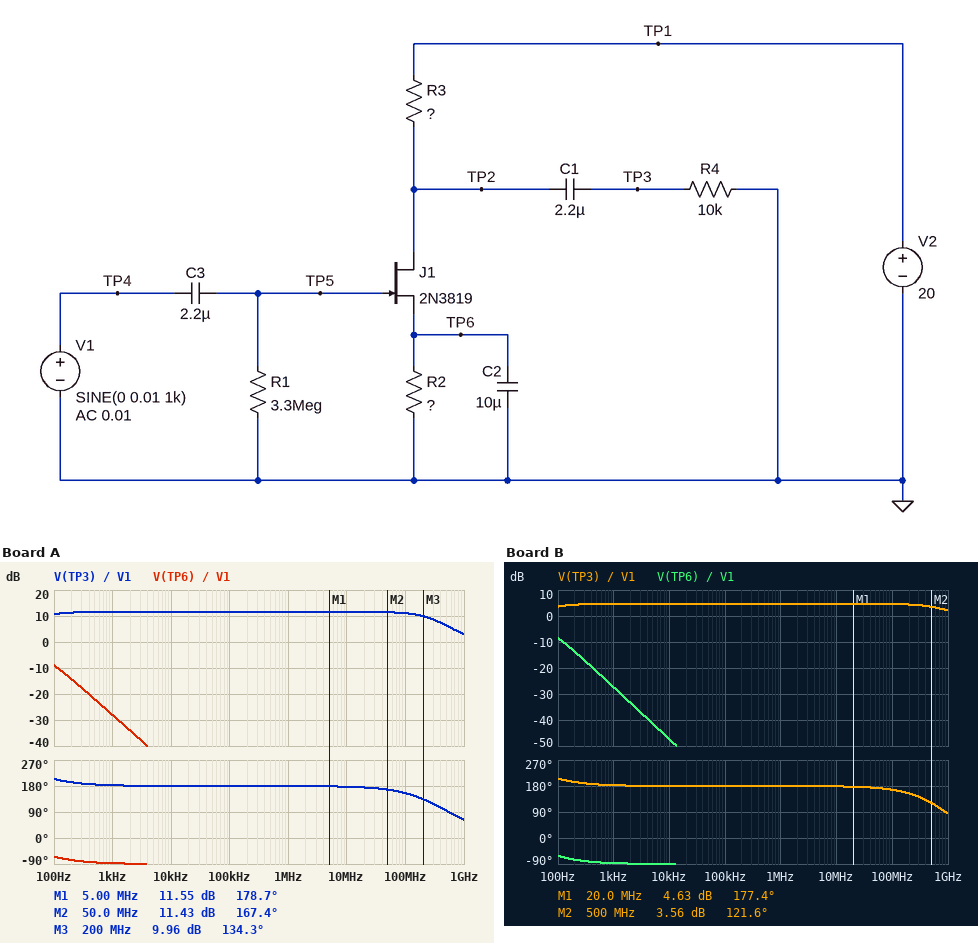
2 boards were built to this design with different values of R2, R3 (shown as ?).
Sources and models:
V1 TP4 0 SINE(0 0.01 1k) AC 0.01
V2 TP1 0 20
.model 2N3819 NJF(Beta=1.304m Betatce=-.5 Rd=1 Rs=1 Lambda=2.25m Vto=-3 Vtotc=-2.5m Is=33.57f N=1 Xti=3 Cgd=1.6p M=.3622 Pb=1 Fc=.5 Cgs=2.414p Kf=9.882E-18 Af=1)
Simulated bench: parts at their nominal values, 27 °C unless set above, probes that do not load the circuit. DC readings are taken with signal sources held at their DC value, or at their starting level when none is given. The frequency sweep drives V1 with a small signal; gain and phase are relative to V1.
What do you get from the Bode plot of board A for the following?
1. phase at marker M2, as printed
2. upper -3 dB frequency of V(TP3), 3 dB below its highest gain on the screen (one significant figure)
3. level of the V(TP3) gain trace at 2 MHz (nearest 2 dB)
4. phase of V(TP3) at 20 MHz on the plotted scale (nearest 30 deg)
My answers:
167.4 deg
300 MHz
12 dB
180 deg
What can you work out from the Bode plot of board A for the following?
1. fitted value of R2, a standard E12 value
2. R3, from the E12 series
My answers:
1.8 kΩ
1.8 kΩ
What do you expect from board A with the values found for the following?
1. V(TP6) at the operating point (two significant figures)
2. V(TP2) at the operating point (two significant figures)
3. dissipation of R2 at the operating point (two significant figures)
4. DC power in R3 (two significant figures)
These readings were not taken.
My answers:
2.1 V
18 V
2.4 mW
2.4 mW
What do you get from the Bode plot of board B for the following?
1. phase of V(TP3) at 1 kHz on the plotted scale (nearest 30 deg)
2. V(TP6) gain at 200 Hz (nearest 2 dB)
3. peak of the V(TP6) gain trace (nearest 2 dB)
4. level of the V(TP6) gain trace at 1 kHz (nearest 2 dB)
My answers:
180 deg
-14 dB
-8 dB
-28 dB
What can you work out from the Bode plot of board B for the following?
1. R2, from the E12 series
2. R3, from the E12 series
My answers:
1.5 kΩ
680 Ω
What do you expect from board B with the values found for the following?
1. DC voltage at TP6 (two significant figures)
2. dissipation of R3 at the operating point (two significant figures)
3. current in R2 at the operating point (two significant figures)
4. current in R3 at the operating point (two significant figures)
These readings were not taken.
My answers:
2.0 V
1.2 mW
1.3 mA
1.3 mA
